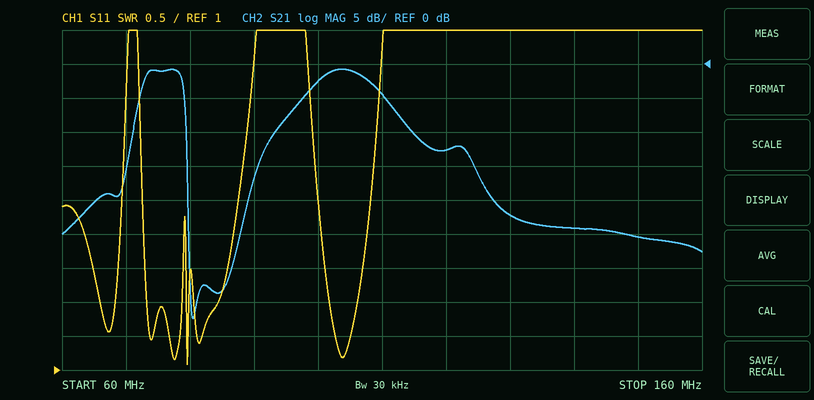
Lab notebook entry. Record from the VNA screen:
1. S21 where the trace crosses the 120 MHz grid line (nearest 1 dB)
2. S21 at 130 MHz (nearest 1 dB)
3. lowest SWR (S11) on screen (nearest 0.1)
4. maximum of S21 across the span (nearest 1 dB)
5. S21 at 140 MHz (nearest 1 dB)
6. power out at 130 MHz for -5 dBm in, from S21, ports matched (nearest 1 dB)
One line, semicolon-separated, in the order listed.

-13 dB; -22 dB; 1.1; -1 dB; -24 dB; -27 dBm
